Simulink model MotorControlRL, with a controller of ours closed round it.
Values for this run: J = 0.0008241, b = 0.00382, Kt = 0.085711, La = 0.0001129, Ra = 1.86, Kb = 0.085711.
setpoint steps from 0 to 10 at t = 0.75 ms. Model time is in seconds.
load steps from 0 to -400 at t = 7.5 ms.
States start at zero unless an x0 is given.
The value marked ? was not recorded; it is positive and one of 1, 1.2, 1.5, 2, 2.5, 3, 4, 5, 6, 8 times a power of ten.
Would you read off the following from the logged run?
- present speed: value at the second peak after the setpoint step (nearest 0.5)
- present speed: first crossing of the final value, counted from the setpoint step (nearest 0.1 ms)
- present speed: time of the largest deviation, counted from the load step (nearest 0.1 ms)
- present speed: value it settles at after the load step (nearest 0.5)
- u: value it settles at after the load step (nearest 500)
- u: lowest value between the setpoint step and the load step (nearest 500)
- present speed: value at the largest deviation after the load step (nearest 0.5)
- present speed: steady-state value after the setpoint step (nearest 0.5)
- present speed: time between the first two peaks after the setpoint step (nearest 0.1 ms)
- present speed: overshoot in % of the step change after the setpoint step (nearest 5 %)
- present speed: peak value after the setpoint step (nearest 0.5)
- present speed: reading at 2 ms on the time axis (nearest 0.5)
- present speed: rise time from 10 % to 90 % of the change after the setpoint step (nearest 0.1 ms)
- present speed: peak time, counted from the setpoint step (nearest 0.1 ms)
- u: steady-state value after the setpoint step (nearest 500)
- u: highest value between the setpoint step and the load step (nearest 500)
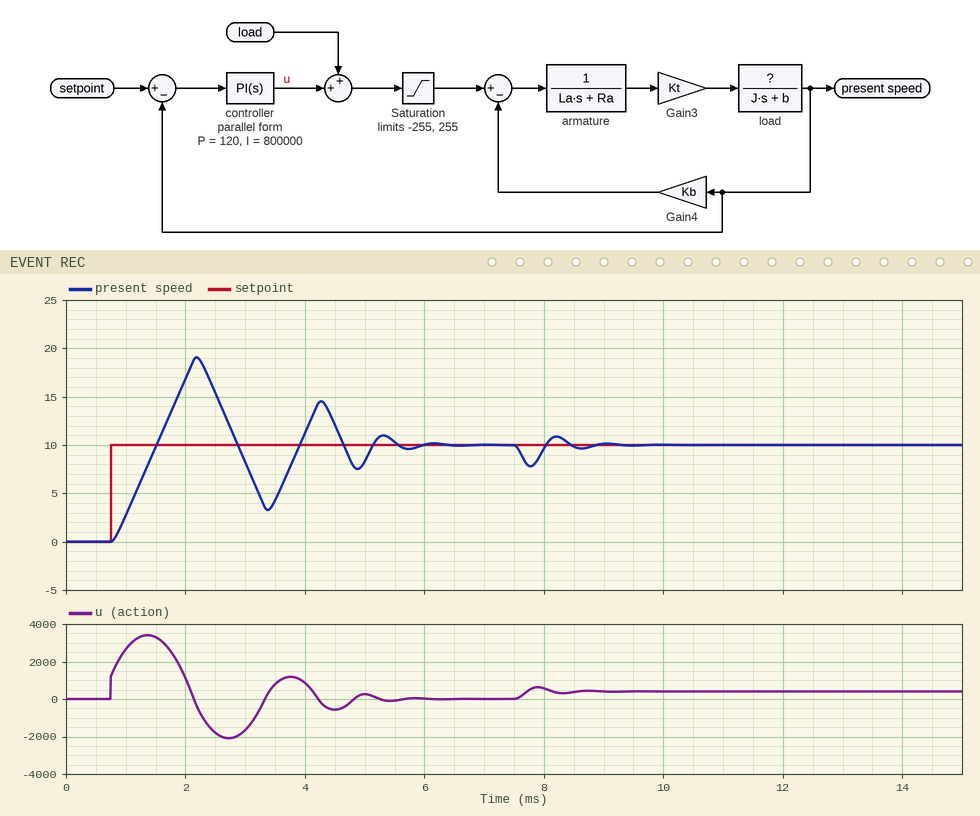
14.5
0.8 ms
0.3 ms
10.0
500
-2000
8.0
10.0
2.1 ms
90 %
19.0
17.0
0.6 ms
1.4 ms
0
3500
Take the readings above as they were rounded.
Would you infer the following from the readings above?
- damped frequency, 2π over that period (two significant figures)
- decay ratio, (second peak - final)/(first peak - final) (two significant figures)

3.0 rad/ms
0.50
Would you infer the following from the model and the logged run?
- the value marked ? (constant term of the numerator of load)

1
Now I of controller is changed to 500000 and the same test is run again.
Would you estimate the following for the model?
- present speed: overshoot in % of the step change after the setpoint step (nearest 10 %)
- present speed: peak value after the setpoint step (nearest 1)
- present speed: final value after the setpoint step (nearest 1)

80 %
18
10
